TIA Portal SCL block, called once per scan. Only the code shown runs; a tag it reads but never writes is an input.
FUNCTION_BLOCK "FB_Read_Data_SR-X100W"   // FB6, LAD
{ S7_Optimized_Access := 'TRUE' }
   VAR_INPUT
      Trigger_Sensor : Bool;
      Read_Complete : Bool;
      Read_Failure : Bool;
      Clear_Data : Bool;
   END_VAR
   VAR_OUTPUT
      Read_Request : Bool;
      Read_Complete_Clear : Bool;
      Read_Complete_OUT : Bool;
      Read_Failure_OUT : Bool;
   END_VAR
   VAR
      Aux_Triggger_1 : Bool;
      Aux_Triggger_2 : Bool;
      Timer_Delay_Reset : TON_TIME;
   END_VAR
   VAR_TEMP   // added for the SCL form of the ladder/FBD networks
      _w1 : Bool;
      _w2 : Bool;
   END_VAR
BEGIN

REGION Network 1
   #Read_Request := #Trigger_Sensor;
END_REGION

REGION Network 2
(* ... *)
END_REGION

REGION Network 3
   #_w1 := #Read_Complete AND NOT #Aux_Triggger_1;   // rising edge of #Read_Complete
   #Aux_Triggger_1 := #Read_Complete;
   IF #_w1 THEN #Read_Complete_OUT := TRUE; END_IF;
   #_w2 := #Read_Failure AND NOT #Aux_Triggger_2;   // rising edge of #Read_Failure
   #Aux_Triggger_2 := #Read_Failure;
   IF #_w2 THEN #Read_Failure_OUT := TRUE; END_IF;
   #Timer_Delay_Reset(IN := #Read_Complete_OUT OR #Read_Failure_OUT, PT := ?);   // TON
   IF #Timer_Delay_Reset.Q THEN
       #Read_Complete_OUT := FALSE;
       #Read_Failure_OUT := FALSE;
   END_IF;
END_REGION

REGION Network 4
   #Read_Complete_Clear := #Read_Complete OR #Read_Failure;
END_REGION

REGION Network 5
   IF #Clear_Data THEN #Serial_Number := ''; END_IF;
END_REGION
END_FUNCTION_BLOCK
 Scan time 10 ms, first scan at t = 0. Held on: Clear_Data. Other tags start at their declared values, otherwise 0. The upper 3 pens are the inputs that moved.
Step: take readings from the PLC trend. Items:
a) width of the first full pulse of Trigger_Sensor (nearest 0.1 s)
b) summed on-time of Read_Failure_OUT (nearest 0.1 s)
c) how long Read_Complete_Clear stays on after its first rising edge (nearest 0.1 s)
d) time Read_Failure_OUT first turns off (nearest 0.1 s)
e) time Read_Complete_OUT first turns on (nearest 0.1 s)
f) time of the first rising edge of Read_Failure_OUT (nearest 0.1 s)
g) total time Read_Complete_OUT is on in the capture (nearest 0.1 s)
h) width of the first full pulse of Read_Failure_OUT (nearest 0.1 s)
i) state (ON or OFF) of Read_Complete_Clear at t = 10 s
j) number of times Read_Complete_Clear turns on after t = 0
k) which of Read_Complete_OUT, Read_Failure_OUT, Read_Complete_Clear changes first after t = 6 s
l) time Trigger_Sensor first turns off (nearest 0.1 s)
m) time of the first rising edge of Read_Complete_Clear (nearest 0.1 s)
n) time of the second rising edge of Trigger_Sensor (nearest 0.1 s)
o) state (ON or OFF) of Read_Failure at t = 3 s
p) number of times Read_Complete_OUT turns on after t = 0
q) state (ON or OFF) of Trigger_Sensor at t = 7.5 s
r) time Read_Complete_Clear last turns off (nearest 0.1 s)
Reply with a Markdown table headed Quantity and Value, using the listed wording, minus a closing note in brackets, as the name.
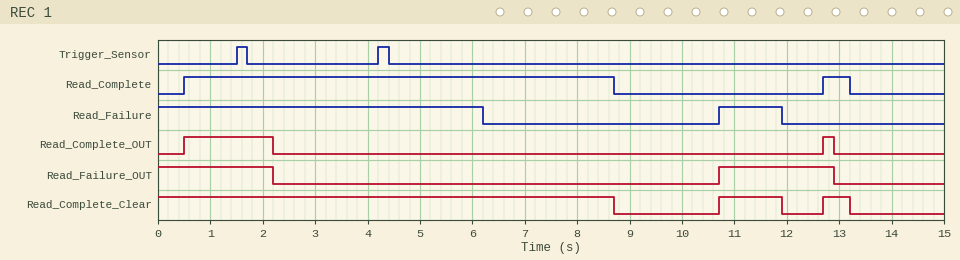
| Quantity | Value |
|---|---|
| width of the first full pulse of Trigger_Sensor | 0.2 s |
| summed on-time of Read_Failure_OUT | 4.4 s |
| how long Read_Complete_Clear stays on after its first rising edge | 1.2 s |
| time Read_Failure_OUT first turns off | 2.2 s |
| time Read_Complete_OUT first turns on | 0.5 s |
| time of the first rising edge of Read_Failure_OUT | 10.7 s |
| total time Read_Complete_OUT is on in the capture | 1.9 s |
| width of the first full pulse of Read_Failure_OUT | 2.2 s |
| state (ON or OFF) of Read_Complete_Clear at t = 10 s | OFF |
| number of times Read_Complete_Clear turns on after t = 0 | 2 |
| which of Read_Complete_OUT, Read_Failure_OUT, Read_Complete_Clear changes first after t = 6 s | Read_Complete_Clear |
| time Trigger_Sensor first turns off | 1.7 s |
| time of the first rising edge of Read_Complete_Clear | 10.7 s |
| time of the second rising edge of Trigger_Sensor | 4.2 s |
| state (ON or OFF) of Read_Failure at t = 3 s | ON |
| number of times Read_Complete_OUT turns on after t = 0 | 2 |
| state (ON or OFF) of Trigger_Sensor at t = 7.5 s | OFF |
| time Read_Complete_Clear last turns off | 13.2 s |
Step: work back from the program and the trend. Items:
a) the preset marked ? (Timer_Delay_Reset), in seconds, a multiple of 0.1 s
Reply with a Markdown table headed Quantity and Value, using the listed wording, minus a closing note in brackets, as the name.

| Quantity | Value |
|---|---|
| the preset marked ? (Timer_Delay_Reset), in seconds, a multiple of 0.1 s | 2.2 s |
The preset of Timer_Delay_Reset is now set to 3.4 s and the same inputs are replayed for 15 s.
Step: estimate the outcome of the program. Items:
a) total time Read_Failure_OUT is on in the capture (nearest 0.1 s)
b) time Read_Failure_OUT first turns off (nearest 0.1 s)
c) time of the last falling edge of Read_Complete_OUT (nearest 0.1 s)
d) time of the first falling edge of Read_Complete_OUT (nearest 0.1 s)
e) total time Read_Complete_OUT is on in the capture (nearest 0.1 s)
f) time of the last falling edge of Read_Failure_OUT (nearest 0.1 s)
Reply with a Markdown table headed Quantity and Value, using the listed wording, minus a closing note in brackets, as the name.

| Quantity | Value |
|---|---|
| total time Read_Failure_OUT is on in the capture | 6.8 s |
| time Read_Failure_OUT first turns off | 3.4 s |
| time of the last falling edge of Read_Complete_OUT | 14.1 s |
| time of the first falling edge of Read_Complete_OUT | 3.4 s |
| total time Read_Complete_OUT is on in the capture | 4.3 s |
| time of the last falling edge of Read_Failure_OUT | 14.1 s |
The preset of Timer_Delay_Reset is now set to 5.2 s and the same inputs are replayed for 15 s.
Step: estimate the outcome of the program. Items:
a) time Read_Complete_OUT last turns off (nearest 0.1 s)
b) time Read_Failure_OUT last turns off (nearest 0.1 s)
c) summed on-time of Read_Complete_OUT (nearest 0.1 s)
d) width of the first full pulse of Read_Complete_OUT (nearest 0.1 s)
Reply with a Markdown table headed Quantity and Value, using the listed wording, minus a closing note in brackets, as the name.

| Quantity | Value |
|---|---|
| time Read_Complete_OUT last turns off | 5.2 s |
| time Read_Failure_OUT last turns off | 5.2 s |
| summed on-time of Read_Complete_OUT | 7.0 s |
| width of the first full pulse of Read_Complete_OUT | 4.7 s |
